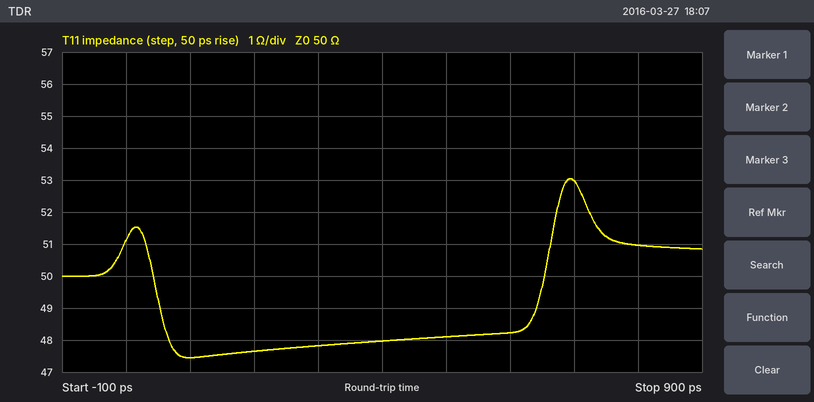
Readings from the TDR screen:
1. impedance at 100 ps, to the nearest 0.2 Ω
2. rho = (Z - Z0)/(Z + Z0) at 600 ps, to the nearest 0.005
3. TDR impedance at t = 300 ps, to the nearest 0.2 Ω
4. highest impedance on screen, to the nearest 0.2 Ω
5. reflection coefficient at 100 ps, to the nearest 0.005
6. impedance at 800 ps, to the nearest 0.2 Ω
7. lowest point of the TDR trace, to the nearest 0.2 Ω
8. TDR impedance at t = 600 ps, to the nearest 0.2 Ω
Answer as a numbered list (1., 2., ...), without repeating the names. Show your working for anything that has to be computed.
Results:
1. 47.4 Ω
2. (48.2 − 50)/(48.2 + 50) ≈ -0.0183, so -0.020 to the nearest 0.005
3. 47.8 Ω
4. 53.0 Ω
5. (47.4 − 50)/(47.4 + 50) ≈ -0.0267, so -0.025 to the nearest 0.005
6. 51.0 Ω
7. 47.4 Ω
8. 48.2 Ω
